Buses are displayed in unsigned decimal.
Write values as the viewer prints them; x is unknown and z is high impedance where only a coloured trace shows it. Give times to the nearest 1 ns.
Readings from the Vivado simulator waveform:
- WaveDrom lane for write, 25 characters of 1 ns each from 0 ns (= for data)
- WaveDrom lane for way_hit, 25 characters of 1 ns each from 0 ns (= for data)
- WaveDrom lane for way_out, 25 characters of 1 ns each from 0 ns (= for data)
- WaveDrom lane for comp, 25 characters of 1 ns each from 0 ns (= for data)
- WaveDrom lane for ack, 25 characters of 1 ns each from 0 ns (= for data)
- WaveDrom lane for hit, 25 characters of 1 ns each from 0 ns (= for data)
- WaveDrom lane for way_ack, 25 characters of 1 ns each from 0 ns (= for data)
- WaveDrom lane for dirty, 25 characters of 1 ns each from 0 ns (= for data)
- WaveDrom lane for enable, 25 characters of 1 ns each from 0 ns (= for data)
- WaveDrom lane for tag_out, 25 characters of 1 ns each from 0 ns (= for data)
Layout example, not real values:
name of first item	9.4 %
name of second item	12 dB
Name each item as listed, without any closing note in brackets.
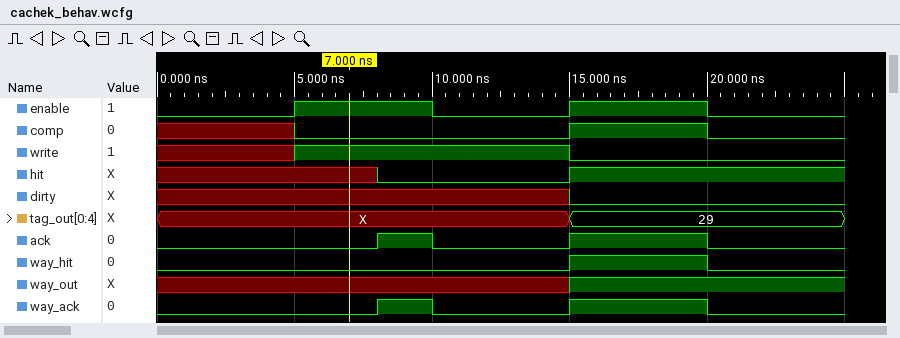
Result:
WaveDrom lane for write, 25 characters of 1 ns each from 0 ns	{name: 'write', wave: 'x....1.........0.........'}
WaveDrom lane for way_hit, 25 characters of 1 ns each from 0 ns	{name: 'way_hit', wave: '0..............1....0....'}
WaveDrom lane for way_out, 25 characters of 1 ns each from 0 ns	{name: 'way_out', wave: 'x..............1.........'}
WaveDrom lane for comp, 25 characters of 1 ns each from 0 ns	{name: 'comp', wave: 'x....0.........1....0....'}
WaveDrom lane for ack, 25 characters of 1 ns each from 0 ns	{name: 'ack', wave: '0.......1.0....1....0....'}
WaveDrom lane for hit, 25 characters of 1 ns each from 0 ns	{name: 'hit', wave: 'x.......0......1.........'}
WaveDrom lane for way_ack, 25 characters of 1 ns each from 0 ns	{name: 'way_ack', wave: '0.......1.0....1....0....'}
WaveDrom lane for dirty, 25 characters of 1 ns each from 0 ns	{name: 'dirty', wave: 'x..............0.........'}
WaveDrom lane for enable, 25 characters of 1 ns each from 0 ns	{name: 'enable', wave: '0....1....0....1....0....'}
WaveDrom lane for tag_out, 25 characters of 1 ns each from 0 ns	{name: 'tag_out', wave: 'x..............=.........', data: '29'}
